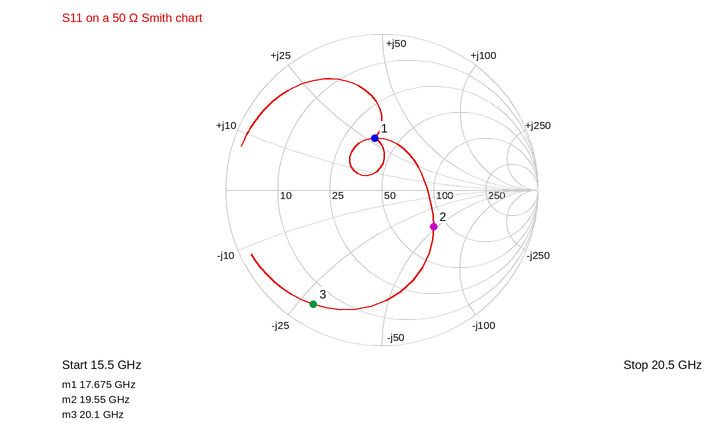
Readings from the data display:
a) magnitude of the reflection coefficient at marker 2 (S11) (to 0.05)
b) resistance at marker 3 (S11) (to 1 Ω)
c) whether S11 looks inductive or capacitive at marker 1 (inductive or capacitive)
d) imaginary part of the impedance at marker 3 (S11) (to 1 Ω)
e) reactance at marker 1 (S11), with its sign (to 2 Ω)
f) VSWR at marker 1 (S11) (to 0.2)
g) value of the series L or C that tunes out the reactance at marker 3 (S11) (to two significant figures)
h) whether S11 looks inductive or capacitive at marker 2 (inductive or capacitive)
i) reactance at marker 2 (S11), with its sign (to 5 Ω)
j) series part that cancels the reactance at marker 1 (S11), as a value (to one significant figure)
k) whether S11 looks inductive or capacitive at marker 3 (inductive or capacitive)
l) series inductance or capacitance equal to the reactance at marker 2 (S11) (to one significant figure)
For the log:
0.40
5 Ω
inductive
-28 Ω
+28 Ω
2.0
220 pH
capacitive
-45 Ω
300 fF
capacitive
200 fF
